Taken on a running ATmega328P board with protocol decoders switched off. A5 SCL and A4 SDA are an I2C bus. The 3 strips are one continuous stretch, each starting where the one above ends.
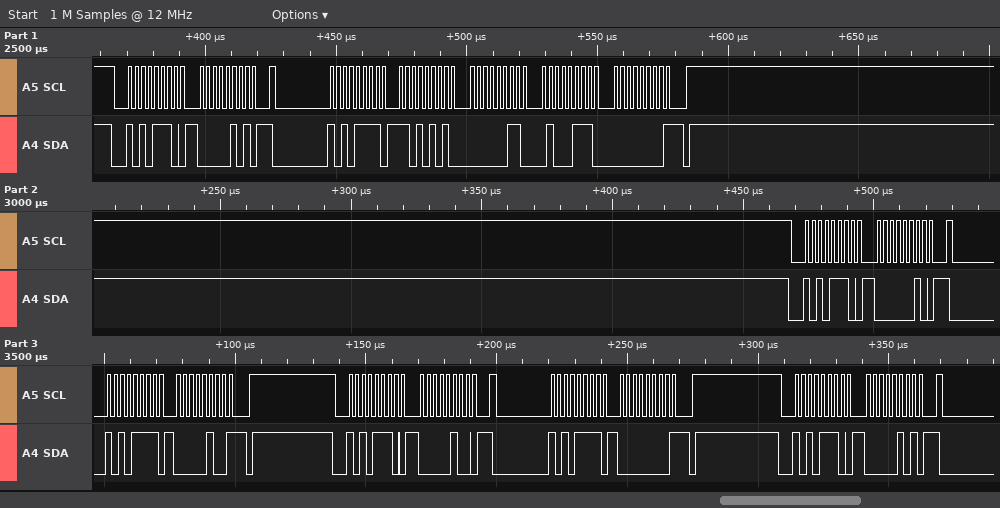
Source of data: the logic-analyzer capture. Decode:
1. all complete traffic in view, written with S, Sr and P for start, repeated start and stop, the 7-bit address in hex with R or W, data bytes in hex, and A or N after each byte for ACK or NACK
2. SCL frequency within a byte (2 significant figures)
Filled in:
S 57W A 05 A Sr 57R A D5 A 03 A 47 A 00 N P S 57W A 02 A Sr 57R A 04 N P S 57W A 04 A Sr 57R A 00 N P S 57W A 05 A
400 kHz
